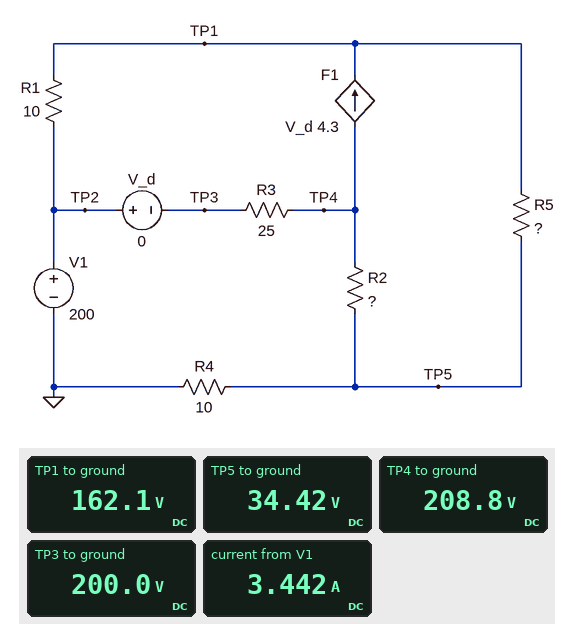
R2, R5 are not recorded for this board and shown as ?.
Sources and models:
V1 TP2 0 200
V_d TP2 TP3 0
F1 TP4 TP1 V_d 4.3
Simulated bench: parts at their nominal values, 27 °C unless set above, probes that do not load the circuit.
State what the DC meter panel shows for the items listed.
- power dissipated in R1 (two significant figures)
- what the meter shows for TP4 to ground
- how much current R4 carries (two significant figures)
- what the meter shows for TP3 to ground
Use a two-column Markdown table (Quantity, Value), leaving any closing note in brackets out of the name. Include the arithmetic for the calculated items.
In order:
| Quantity | Value |
|---|---|
| power dissipated in R1 | (200 V - 162.1 V)^2 / 10 Ω = 140 W |
| what the meter shows for TP4 to ground | 208.8 V |
| how much current R4 carries | (34.42 V) / 10 Ω = 3.4 A |
| what the meter shows for TP3 to ground | 200.0 V |
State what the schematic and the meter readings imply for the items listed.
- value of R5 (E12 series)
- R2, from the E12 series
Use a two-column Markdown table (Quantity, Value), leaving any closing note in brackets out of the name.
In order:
| Quantity | Value |
|---|---|
| value of R5 | 56 Ω |
| R2, from the E12 series | 150 Ω |
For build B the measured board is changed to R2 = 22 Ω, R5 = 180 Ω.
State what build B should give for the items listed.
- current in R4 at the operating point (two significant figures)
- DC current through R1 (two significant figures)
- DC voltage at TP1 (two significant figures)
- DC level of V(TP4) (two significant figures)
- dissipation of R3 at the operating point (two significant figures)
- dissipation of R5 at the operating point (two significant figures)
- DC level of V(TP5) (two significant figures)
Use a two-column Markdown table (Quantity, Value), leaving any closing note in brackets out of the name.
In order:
| Quantity | Value |
|---|---|
| current in R4 at the operating point | 8.2 A |
| DC current through R1 | 11 A |
| DC voltage at TP1 | 93 V |
| DC level of V(TP4) | 260 V |
| dissipation of R3 at the operating point | 150 W |
| dissipation of R5 at the operating point | 650 mW |
| DC level of V(TP5) | 82 V |
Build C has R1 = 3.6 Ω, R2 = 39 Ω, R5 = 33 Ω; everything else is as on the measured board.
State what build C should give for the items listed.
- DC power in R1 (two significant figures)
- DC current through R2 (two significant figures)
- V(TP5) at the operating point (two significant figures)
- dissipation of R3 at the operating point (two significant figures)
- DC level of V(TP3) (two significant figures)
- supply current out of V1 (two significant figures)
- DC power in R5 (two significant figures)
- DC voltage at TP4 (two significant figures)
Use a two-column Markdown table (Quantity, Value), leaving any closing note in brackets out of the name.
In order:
| Quantity | Value |
|---|---|
| DC power in R1 | 250 W |
| DC current through R2 | 4.1 A |
| V(TP5) at the operating point | 71 V |
| dissipation of R3 at the operating point | 39 W |
| DC level of V(TP3) | 200 V |
| supply current out of V1 | 7.1 A |
| DC power in R5 | 300 W |
| DC voltage at TP4 | 230 V |
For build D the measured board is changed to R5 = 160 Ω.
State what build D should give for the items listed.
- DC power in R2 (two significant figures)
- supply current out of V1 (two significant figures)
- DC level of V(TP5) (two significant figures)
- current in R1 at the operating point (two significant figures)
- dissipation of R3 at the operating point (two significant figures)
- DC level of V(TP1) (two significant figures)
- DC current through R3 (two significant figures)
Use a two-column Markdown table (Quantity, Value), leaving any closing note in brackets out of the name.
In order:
| Quantity | Value |
|---|---|
| DC power in R2 | 230 W |
| supply current out of V1 | 2.2 A |
| DC level of V(TP5) | 22 V |
| current in R1 at the operating point | 2.6 A |
| dissipation of R3 at the operating point | 3.6 W |
| DC level of V(TP1) | 170 V |
| DC current through R3 | 380 mA |
